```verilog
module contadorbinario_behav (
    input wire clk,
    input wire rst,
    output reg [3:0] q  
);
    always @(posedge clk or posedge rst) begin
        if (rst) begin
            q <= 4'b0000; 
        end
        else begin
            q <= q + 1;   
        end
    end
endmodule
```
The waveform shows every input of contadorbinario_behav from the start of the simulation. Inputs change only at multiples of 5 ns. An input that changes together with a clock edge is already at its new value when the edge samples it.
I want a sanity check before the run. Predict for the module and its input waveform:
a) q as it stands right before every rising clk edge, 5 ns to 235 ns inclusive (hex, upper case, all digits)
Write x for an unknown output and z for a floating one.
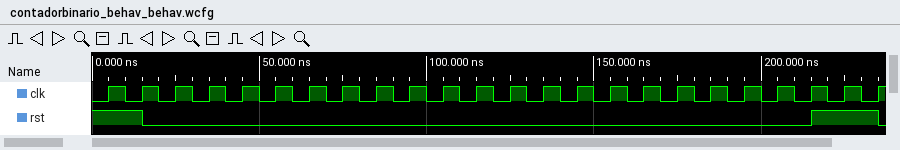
0, 0, 1, 2, 3, 4, 5, 6, 7, 8, 9, A, B, C, D, E, F, 0, 1, 2, 3, 4, 0, 0
